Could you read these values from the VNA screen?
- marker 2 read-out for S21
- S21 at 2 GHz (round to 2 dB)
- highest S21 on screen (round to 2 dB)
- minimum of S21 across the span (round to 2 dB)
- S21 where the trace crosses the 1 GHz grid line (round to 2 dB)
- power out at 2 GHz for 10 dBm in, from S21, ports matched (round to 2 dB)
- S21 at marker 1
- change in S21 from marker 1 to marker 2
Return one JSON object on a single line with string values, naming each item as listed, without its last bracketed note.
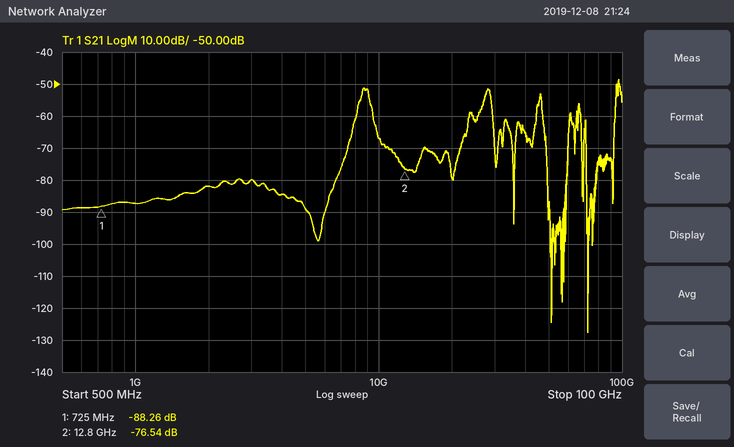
{"marker 2 read-out for S21": "-76.54 dB", "S21 at 2 GHz": "-82 dB", "highest S21 on screen": "-48 dB", "minimum of S21 across the span": "-128 dB", "S21 where the trace crosses the 1 GHz grid line": "-88 dB", "power out at 2 GHz for 10 dBm in, from S21, ports matched": "-72 dBm", "S21 at marker 1": "-88.26 dB", "change in S21 from marker 1 to marker 2": "11.72 dB"}
